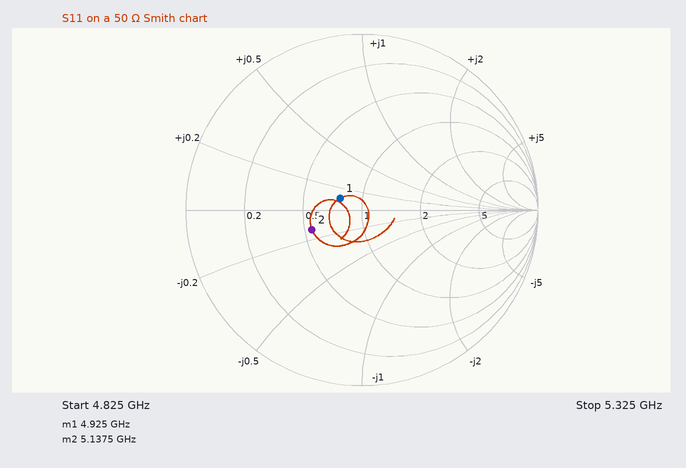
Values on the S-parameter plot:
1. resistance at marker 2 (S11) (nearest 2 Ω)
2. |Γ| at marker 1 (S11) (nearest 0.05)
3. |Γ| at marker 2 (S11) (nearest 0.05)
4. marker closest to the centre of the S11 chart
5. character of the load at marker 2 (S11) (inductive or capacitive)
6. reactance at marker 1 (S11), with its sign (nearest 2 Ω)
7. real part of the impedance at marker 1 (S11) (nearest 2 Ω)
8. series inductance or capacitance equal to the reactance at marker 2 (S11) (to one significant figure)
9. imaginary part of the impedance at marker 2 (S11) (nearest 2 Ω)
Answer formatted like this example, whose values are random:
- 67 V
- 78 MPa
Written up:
- 28 Ω
- 0.15
- 0.30
- marker 1
- capacitive
- +6 Ω
- 38 Ω
- 5 pF
- -6 Ω
